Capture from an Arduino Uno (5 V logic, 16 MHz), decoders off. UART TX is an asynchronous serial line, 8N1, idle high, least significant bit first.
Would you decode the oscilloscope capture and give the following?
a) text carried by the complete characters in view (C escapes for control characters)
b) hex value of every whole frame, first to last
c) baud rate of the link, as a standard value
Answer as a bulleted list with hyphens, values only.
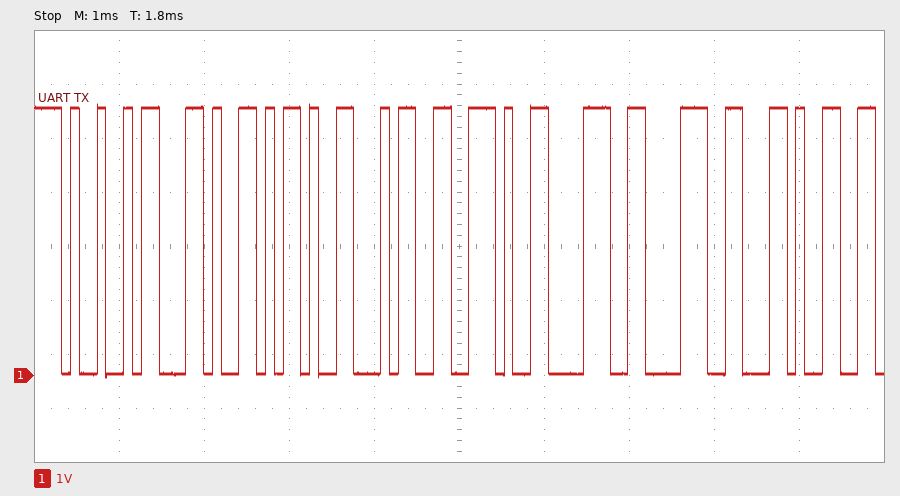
- "I,-4.88,"
- 0x49 0x2C 0x2D 0x34 0x2E 0x38 0x38 0x2C
- 9600 baud
